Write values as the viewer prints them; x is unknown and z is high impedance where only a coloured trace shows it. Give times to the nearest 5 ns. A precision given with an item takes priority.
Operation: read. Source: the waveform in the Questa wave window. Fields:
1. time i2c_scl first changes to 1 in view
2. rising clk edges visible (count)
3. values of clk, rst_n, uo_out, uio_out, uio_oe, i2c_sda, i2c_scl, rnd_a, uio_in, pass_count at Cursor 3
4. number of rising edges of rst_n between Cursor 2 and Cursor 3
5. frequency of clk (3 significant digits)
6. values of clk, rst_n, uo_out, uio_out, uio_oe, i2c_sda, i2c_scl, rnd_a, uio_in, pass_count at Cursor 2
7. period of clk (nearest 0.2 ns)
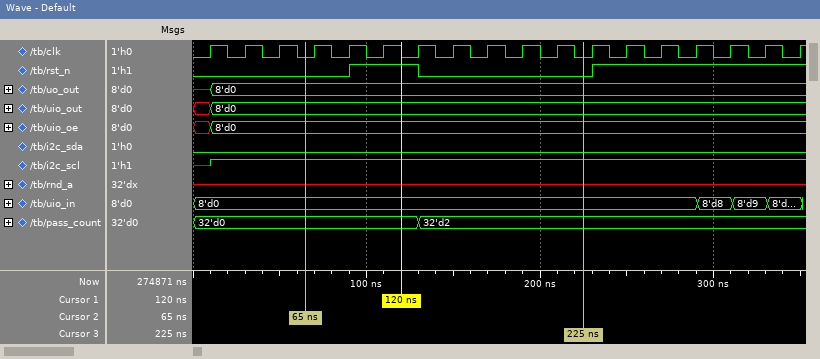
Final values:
10 ns
18
clk=0, rst_n=0, uo_out=8'd0, uio_out=8'd0, uio_oe=8'd0, i2c_sda=0, i2c_scl=1, rnd_a=x, uio_in=8'd0, pass_count=32'd2
1
50.0 MHz
clk=0, rst_n=0, uo_out=8'd0, uio_out=8'd0, uio_oe=8'd0, i2c_sda=0, i2c_scl=1, rnd_a=x, uio_in=8'd0, pass_count=32'd0
20 ns
